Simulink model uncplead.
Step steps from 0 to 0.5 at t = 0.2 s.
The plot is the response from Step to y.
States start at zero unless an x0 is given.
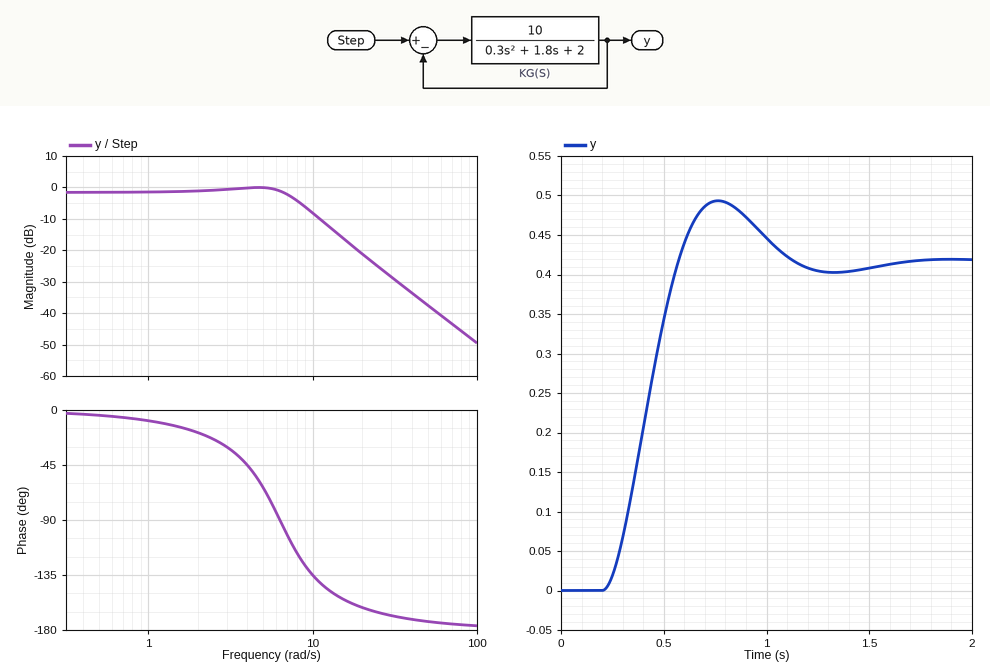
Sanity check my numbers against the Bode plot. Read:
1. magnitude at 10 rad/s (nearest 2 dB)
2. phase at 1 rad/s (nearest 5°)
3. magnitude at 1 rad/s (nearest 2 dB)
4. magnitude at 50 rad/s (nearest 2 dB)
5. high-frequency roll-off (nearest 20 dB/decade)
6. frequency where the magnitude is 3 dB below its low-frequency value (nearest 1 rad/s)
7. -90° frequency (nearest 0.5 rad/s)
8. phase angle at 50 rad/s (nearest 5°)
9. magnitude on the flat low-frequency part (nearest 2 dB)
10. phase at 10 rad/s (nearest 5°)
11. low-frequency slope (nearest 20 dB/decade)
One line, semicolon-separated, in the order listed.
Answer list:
-8 dB; -10°; -2 dB; -38 dB; -40 dB/decade; 8 rad/s; 6.5 rad/s; -175°; -2 dB; -135°; 0 dB/decade
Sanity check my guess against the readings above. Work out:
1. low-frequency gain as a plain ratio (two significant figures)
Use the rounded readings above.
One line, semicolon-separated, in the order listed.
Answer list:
0.79
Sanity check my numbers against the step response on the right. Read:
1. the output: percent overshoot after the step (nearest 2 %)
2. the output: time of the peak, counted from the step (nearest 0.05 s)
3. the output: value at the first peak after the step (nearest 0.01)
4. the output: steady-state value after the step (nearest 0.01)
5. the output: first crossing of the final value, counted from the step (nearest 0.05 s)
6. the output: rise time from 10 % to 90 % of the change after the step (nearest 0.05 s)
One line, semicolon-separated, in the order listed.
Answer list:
18 %; 0.55 s; 0.49; 0.42; 0.35 s; 0.25 s
